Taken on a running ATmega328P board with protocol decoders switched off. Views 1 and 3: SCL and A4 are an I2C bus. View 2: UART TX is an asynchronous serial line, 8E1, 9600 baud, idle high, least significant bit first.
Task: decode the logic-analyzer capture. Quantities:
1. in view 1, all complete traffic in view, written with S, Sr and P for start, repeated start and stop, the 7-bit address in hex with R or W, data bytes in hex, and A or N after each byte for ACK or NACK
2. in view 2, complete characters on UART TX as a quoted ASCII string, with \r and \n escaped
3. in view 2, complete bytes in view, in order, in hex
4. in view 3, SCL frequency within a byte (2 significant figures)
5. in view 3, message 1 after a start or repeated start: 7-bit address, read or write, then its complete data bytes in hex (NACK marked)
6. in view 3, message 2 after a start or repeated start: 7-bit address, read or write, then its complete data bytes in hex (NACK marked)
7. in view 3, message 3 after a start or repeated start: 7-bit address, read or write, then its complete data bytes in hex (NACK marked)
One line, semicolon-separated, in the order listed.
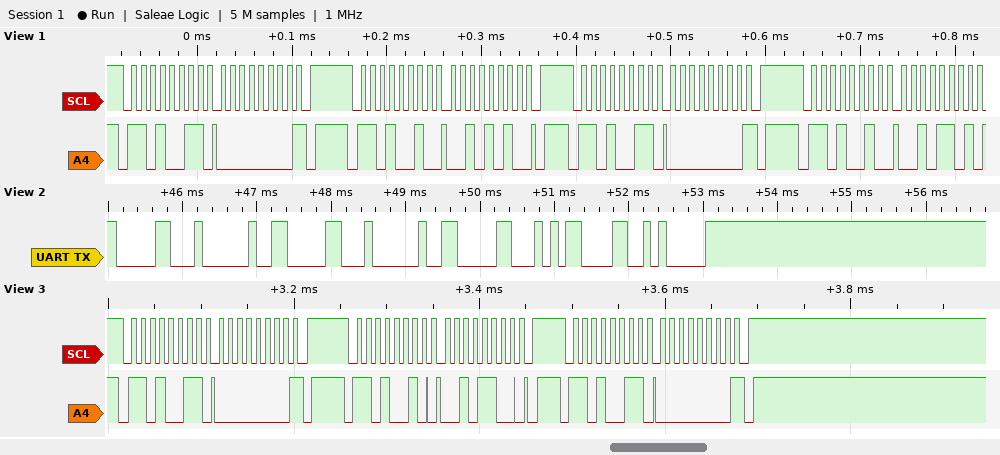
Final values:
S 69R A 00 N P S 69W A 2A A P S 69R A 00 N P S 69W A 2D A; "0 0 0\r\n"; 0x30 0x20 0x30 0x20 0x30 0x0D 0x0A; 100 kHz; 0x69 read: 00 NACK; 0x69 write: 2C; 0x69 read: 00 NACK
